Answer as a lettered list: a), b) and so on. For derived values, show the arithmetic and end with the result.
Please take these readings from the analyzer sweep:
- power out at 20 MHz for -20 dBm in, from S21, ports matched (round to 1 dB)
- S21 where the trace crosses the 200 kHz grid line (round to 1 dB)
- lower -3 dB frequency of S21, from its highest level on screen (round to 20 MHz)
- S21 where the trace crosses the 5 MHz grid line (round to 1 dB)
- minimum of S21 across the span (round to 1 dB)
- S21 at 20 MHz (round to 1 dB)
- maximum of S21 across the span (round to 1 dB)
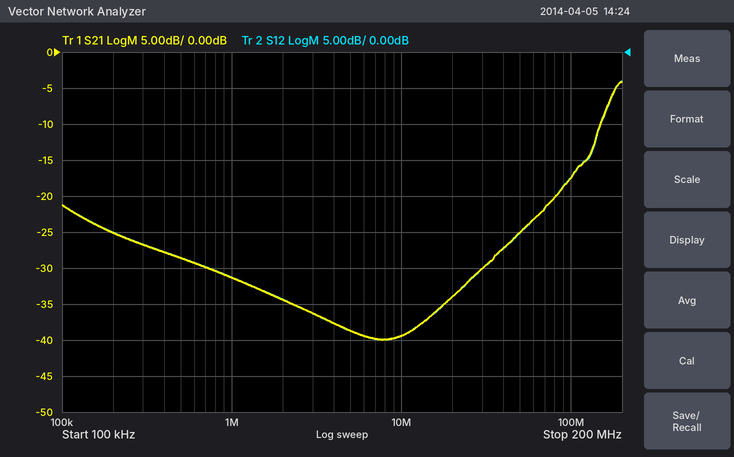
a) -20 dBm + (-34 dB) = -54 dBm
b) -25 dB
c) 160 MHz
d) -39 dB
e) -40 dB
f) -34 dB
g) -4 dB
